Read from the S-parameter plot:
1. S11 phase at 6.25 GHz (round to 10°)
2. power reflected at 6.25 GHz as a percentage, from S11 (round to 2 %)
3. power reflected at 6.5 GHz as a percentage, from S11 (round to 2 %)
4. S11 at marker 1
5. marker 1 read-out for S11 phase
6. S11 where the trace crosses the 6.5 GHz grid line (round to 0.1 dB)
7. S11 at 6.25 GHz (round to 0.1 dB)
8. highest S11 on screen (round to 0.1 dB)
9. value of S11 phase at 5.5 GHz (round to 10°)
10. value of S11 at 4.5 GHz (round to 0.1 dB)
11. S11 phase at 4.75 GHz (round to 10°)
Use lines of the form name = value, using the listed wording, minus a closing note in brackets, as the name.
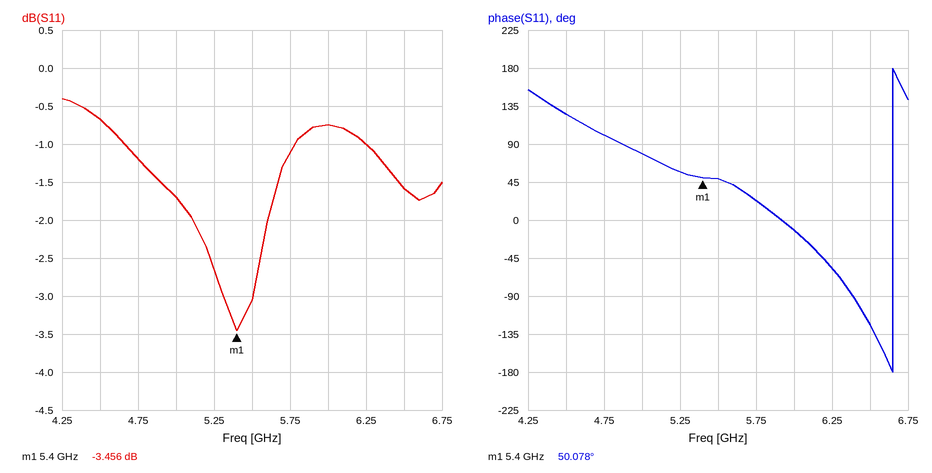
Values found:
S11 phase at 6.25 GHz = -60°
power reflected at 6.25 GHz as a percentage, from S11 = 80 %
power reflected at 6.5 GHz as a percentage, from S11 = 70 %
S11 at marker 1 = -3.456 dB
marker 1 read-out for S11 phase = 50.078°
S11 where the trace crosses the 6.5 GHz grid line = -1.6 dB
S11 at 6.25 GHz = -1.0 dB
highest S11 on screen = -0.4 dB
value of S11 phase at 5.5 GHz = 50°
value of S11 at 4.5 GHz = -0.7 dB
S11 phase at 4.75 GHz = 100°
